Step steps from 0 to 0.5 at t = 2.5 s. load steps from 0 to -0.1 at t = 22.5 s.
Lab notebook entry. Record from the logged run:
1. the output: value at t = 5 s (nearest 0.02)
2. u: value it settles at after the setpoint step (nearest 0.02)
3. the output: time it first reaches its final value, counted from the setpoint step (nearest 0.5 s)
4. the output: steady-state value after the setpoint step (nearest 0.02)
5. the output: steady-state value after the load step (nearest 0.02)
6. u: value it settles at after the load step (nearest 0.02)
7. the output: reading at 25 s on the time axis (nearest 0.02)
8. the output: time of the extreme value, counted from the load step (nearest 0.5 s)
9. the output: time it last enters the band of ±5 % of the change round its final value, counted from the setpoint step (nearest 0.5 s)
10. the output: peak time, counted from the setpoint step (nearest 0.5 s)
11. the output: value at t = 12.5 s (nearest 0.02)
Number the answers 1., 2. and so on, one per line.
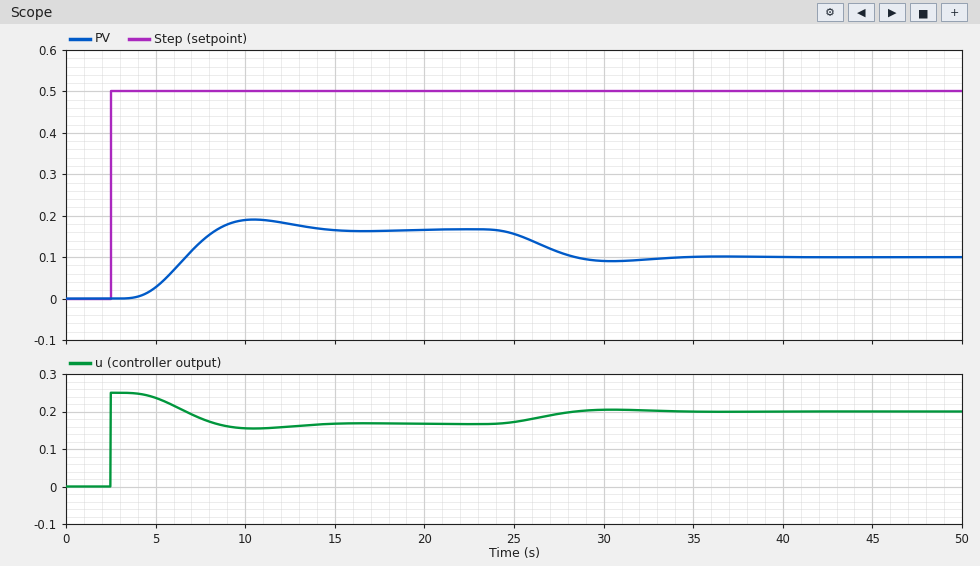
1. 0.02
2. 0.16
3. 6.0 s
4. 0.16
5. 0.10
6. 0.20
7. 0.16
8. 8.0 s
9. 10.5 s
10. 8.0 s
11. 0.18
